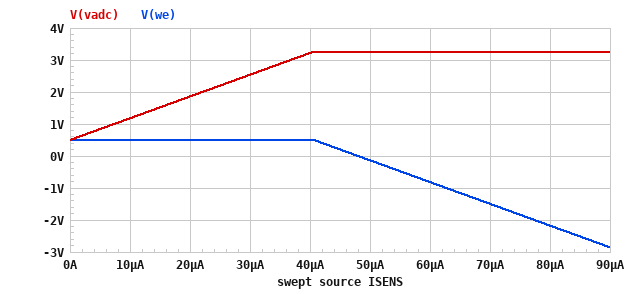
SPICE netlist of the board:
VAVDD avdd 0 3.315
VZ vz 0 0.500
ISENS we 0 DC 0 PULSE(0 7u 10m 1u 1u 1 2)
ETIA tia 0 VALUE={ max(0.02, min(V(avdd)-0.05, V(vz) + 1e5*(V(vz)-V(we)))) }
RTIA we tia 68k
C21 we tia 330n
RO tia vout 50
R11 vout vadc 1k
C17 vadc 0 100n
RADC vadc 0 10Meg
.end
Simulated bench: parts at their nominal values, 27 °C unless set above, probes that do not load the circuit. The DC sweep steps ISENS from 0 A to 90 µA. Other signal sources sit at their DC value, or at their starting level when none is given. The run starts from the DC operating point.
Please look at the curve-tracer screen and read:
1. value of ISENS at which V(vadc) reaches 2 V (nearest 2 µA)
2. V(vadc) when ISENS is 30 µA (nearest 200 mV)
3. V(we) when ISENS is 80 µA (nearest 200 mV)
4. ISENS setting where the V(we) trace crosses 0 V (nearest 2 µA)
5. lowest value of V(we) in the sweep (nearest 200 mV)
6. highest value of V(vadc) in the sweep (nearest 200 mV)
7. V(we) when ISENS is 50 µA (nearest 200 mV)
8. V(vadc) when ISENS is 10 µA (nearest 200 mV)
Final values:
22 µA
2.6 V
-2.2 V
48 µA
-2.8 V
3.2 V
-200 mV
1.2 V
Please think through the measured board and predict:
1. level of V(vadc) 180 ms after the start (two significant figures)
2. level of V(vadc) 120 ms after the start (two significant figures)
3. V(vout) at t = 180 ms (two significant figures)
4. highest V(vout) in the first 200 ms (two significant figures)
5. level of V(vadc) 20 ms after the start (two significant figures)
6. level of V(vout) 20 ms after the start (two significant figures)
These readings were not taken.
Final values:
980 mV
970 mV
980 mV
980 mV
670 mV
670 mV
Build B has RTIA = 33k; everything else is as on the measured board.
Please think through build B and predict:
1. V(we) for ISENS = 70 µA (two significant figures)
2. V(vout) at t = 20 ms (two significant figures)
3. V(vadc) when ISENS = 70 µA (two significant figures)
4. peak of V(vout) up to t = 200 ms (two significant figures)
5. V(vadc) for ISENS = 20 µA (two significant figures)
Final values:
500 mV
640 mV
2.8 V
730 mV
1.2 V
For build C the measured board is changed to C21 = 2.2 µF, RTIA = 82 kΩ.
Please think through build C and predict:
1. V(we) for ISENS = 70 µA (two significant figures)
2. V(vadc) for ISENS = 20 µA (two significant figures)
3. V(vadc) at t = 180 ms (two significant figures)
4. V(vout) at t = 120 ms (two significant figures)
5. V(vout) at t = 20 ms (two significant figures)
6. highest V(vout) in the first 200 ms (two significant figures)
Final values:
-2.5 V
2.1 V
850 mV
760 mV
530 mV
870 mV
